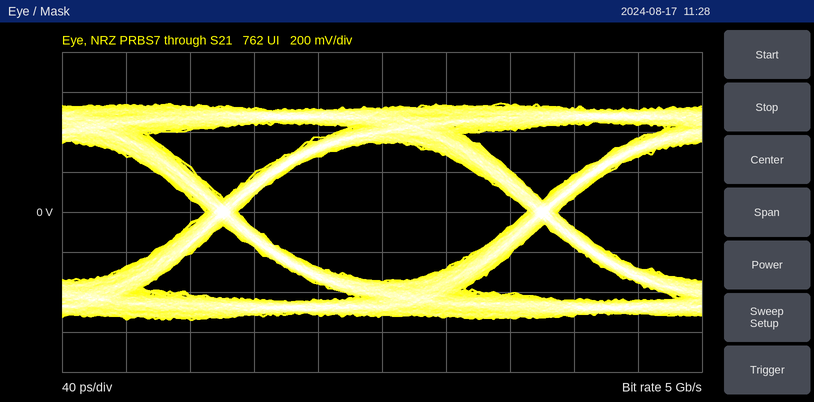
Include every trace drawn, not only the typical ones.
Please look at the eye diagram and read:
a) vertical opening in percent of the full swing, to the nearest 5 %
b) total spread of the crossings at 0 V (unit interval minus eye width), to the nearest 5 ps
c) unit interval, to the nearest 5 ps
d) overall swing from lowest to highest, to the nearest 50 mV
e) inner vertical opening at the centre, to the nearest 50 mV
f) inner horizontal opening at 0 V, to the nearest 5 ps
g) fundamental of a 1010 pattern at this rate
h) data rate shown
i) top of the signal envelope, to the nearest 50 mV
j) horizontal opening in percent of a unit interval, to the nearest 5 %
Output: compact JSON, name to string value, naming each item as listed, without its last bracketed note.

{"vertical opening in percent of the full swing, to the nearest 5 %": "65 %", "total spread of the crossings at 0 V (unit interval minus eye width), to the nearest 5 ps": "20 ps", "unit interval, to the nearest 5 ps": "200 ps", "overall swing from lowest to highest, to the nearest 50 mV": "1.10 V", "inner vertical opening at the centre, to the nearest 50 mV": "700 mV", "inner horizontal opening at 0 V, to the nearest 5 ps": "180 ps", "fundamental of a 1010 pattern at this rate": "2.5 GHz", "data rate shown": "5 Gb/s", "top of the signal envelope, to the nearest 50 mV": "550 mV", "horizontal opening in percent of a unit interval, to the nearest 5 %": "90 %"}
